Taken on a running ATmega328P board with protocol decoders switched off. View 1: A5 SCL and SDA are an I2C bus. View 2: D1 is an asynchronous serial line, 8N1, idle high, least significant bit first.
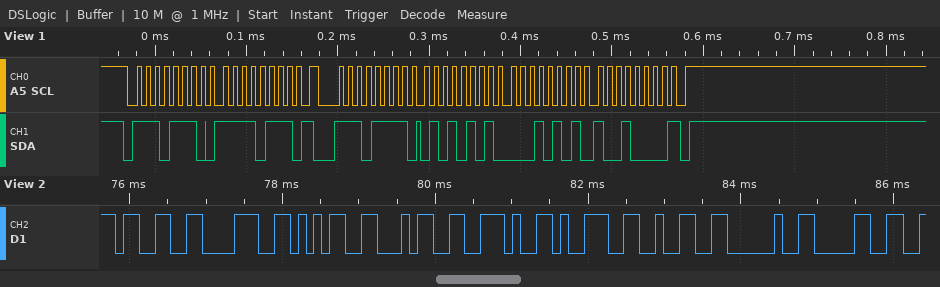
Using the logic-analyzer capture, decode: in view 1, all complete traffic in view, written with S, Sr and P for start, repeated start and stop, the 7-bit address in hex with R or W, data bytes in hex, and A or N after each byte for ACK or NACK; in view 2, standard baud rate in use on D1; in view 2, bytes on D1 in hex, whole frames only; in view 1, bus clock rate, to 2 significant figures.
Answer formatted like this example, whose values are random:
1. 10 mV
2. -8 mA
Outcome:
1. S 77W A F7 A Sr 77R A 55 A 15 A 90 N P
2. 9600 baud
3. 33 38 35 34 2E 39 32 20 30
4. 100 kHz
